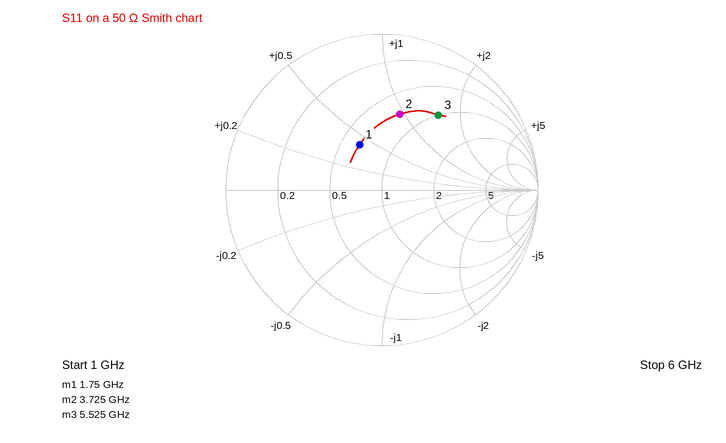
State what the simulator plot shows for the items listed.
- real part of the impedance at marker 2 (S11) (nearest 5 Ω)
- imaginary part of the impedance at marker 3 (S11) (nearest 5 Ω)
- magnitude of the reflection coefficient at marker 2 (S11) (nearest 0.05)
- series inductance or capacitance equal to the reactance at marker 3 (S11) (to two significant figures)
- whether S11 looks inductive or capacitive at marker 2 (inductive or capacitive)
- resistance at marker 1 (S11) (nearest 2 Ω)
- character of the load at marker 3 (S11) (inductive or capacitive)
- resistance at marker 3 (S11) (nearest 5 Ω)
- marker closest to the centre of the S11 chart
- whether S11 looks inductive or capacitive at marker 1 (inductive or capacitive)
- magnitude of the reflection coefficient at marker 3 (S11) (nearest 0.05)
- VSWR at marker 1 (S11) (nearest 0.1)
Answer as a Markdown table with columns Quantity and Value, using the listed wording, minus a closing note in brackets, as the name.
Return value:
| Quantity | Value |
|---|---|
| real part of the impedance at marker 2 (S11) | 35 Ω |
| imaginary part of the impedance at marker 3 (S11) | +75 Ω |
| magnitude of the reflection coefficient at marker 2 (S11) | 0.50 |
| series inductance or capacitance equal to the reactance at marker 3 (S11) | 2.2 nH |
| whether S11 looks inductive or capacitive at marker 2 | inductive |
| resistance at marker 1 (S11) | 32 Ω |
| character of the load at marker 3 (S11) | inductive |
| resistance at marker 3 (S11) | 50 Ω |
| marker closest to the centre of the S11 chart | marker 1 |
| whether S11 looks inductive or capacitive at marker 1 | inductive |
| magnitude of the reflection coefficient at marker 3 (S11) | 0.60 |
| VSWR at marker 1 (S11) | 2.0 |
